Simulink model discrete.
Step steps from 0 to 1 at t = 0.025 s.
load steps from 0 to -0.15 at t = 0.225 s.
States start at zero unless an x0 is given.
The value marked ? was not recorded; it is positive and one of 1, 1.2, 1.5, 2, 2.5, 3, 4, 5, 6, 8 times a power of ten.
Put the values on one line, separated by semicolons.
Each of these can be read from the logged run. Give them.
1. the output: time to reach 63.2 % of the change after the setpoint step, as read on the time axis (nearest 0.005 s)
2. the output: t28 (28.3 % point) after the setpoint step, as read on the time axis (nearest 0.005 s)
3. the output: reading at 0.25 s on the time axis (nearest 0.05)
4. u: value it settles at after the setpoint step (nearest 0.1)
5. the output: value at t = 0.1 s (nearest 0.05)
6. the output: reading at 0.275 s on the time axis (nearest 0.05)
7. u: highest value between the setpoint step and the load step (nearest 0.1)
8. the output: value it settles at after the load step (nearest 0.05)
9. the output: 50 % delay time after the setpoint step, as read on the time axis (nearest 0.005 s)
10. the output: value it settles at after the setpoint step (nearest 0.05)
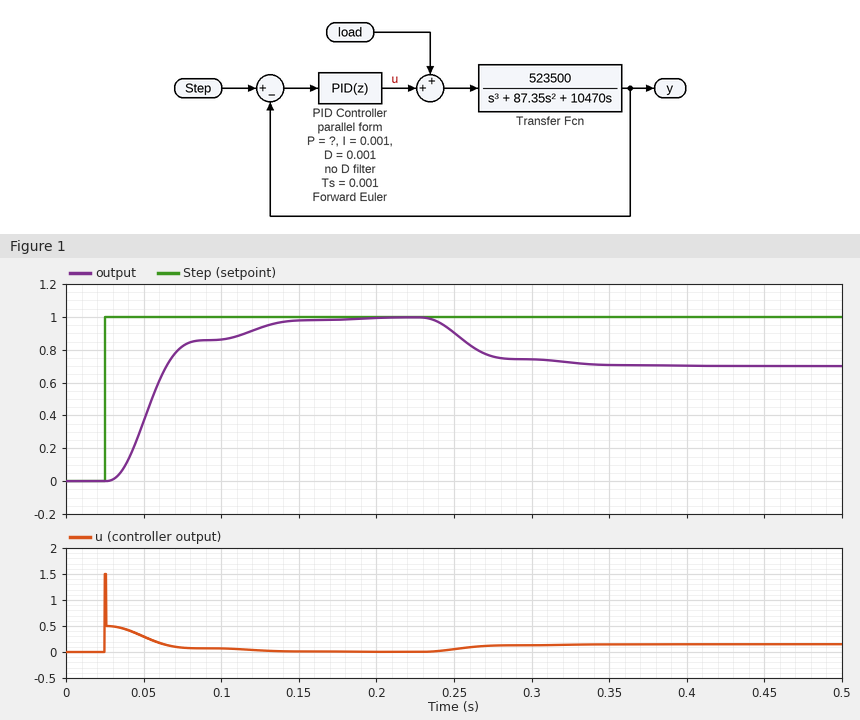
0.060 s; 0.045 s; 0.90; 0.0; 0.85; 0.75; 1.5; 0.70; 0.055 s; 1.00
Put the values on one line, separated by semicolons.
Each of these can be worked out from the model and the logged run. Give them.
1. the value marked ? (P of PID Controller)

0.5
